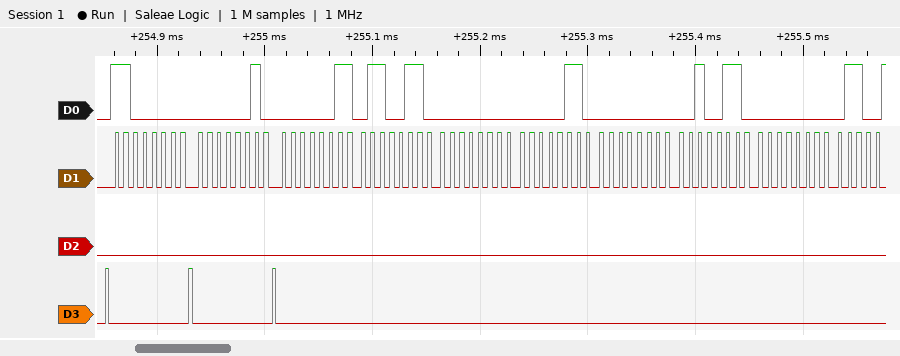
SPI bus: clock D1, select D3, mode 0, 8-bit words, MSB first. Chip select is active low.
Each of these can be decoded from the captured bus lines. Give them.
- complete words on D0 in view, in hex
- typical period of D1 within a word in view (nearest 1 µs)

C0, 02, 03, 66, 00, 06, 00, 26, 00
9 µs
